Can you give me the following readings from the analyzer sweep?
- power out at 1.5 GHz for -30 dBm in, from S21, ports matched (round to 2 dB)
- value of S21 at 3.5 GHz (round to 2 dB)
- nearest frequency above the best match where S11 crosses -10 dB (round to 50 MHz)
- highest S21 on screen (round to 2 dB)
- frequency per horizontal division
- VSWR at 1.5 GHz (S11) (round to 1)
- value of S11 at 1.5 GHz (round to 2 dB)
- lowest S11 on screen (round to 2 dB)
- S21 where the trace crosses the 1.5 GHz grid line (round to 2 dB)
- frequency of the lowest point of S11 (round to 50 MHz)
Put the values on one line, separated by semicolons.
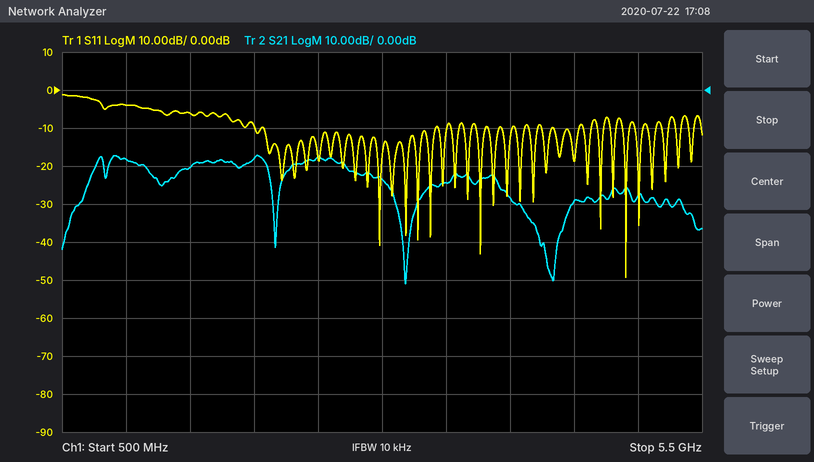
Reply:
-50 dBm; -24 dB; 4.95 GHz; -18 dB; 500 MHz; 3; -6 dB; -50 dB; -20 dB; 4.90 GHz
